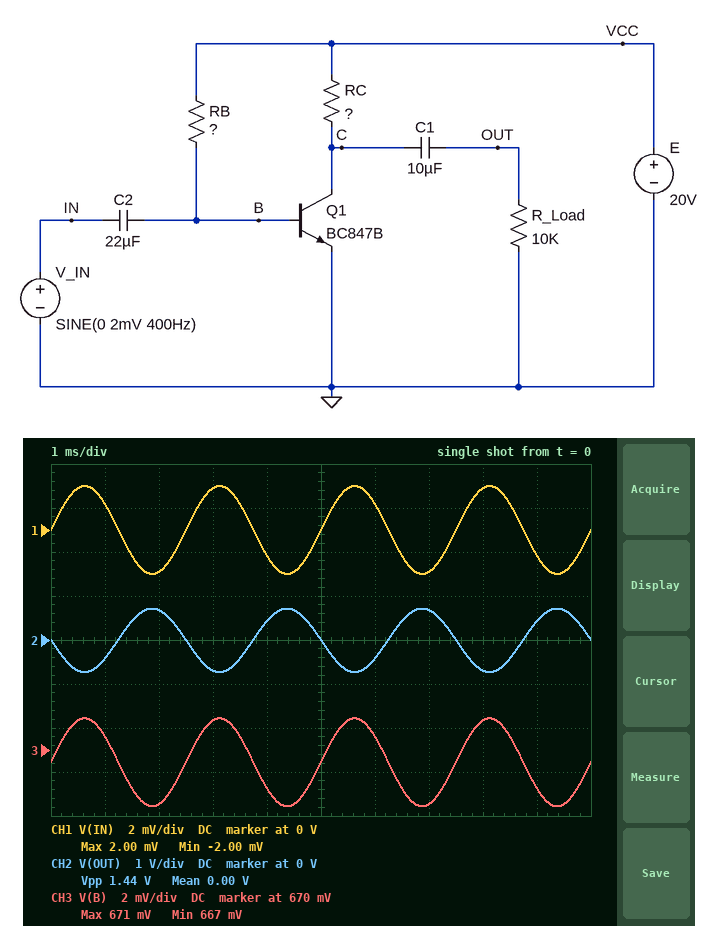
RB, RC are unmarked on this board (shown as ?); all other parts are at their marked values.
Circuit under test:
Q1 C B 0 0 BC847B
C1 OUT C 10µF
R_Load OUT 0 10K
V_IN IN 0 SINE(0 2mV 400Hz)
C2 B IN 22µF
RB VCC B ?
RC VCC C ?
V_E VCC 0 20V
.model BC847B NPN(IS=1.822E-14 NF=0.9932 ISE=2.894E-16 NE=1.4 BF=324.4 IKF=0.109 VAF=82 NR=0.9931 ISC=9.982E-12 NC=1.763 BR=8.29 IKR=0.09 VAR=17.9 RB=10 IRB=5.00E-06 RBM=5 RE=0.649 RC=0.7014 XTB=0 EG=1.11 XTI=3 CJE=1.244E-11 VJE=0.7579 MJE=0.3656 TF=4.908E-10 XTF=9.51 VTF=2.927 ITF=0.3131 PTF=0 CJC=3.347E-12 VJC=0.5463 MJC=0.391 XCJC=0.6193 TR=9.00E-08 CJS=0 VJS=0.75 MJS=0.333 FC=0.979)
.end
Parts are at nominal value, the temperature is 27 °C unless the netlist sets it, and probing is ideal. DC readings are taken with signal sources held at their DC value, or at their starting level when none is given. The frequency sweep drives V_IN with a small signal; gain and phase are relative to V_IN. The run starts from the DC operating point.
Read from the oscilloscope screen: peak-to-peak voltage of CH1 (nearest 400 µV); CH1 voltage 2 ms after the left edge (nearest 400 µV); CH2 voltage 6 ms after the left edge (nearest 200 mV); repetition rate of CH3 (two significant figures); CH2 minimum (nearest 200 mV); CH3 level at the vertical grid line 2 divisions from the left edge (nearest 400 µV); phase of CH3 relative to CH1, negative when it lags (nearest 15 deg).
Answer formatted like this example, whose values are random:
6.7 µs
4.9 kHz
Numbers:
4.0 mV
-2.0 mV
-400 mV
400 Hz
-800 mV
667.6 mV
0 deg
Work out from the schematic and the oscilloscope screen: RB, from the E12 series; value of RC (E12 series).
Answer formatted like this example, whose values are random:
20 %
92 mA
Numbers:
1.8 MΩ
5.6 kΩ
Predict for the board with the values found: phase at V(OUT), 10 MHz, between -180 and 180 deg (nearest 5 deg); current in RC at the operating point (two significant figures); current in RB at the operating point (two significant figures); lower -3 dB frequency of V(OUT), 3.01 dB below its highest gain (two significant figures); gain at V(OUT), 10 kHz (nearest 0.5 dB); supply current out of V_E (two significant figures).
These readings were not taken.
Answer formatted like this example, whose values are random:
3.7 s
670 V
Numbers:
145 deg
3.3 mA
11 µA
3.2 Hz
51.0 dB
3.3 mA
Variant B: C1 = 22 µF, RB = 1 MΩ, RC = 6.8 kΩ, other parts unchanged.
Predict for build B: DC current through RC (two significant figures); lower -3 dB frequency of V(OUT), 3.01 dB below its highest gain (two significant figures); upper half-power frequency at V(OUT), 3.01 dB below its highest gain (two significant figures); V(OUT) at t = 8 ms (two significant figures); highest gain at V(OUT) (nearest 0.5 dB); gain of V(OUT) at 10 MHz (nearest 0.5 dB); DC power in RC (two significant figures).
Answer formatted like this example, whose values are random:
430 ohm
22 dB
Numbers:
2.9 mA
89 Hz
1.2 MHz
-35 mV
31.0 dB
12.5 dB
58 mW
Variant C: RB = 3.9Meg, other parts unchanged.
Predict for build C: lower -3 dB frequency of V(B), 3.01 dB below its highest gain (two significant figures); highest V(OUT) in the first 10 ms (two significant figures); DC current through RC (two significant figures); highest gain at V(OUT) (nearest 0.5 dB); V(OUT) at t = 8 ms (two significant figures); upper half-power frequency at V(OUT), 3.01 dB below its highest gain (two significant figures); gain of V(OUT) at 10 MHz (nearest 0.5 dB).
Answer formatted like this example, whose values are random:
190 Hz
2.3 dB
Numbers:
1.3 Hz
410 mV
1.7 mA
46.5 dB
-410 mV
34 MHz
46.0 dB
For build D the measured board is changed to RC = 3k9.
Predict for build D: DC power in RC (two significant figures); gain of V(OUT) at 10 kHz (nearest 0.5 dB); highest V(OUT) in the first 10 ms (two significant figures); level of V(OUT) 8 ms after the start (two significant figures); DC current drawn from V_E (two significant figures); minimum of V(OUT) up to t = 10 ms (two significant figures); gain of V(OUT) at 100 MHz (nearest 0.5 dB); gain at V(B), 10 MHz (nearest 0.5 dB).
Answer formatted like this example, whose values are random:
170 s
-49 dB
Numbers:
47 mW
49.5 dB
600 mV
-590 mV
3.5 mA
-620 mV
39.0 dB
0 dB
